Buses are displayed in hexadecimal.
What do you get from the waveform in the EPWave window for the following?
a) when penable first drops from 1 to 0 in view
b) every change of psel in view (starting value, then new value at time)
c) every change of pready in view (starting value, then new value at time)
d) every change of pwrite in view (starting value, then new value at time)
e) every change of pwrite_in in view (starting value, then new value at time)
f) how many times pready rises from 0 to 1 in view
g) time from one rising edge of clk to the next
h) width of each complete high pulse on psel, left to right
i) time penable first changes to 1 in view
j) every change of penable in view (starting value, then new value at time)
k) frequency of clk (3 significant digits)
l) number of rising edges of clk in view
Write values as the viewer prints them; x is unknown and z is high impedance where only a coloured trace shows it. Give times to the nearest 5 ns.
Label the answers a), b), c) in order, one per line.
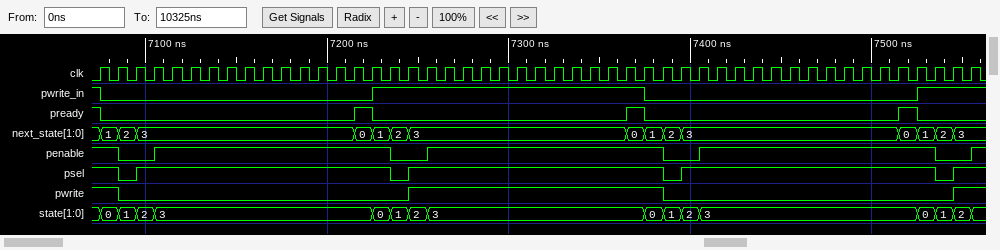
a) 7085 ns
b) 1, 0 at 7085 ns, 1 at 7095 ns, 0 at 7235 ns, 1 at 7245 ns, 0 at 7385 ns, 1 at 7395 ns, 0 at 7535 ns, 1 at 7545 ns
c) 1, 0 at 7075 ns, 1 at 7215 ns, 0 at 7225 ns, 1 at 7365 ns, 0 at 7375 ns, 1 at 7515 ns, 0 at 7525 ns
d) 1, 0 at 7085 ns, 1 at 7245 ns, 0 at 7385 ns, 1 at 7545 ns
e) 1, 0 at 7075 ns, 1 at 7225 ns, 0 at 7375 ns, 1 at 7525 ns
f) 3
g) 10 ns
h) 140 ns, 140 ns, 140 ns
i) 7105 ns
j) 1, 0 at 7085 ns, 1 at 7105 ns, 0 at 7235 ns, 1 at 7255 ns, 0 at 7385 ns, 1 at 7405 ns, 0 at 7535 ns, 1 at 7555 ns
k) 100 MHz
l) 49
